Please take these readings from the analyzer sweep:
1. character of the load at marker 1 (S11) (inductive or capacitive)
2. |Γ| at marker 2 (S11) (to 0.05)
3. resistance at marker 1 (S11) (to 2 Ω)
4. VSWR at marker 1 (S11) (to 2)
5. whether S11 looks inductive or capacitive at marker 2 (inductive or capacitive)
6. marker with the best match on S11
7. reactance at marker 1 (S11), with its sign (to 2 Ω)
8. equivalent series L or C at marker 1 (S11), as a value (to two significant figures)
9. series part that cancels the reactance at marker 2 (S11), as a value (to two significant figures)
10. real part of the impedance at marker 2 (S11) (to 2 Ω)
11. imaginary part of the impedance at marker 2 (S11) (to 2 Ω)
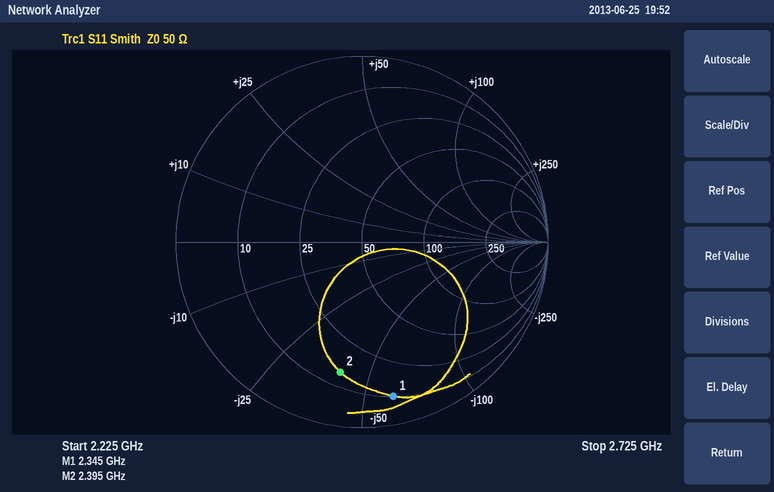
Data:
capacitive
0.70
10 Ω
12
capacitive
marker 2
-60 Ω
1.1 pF
2.7 nH
14 Ω
-40 Ω
